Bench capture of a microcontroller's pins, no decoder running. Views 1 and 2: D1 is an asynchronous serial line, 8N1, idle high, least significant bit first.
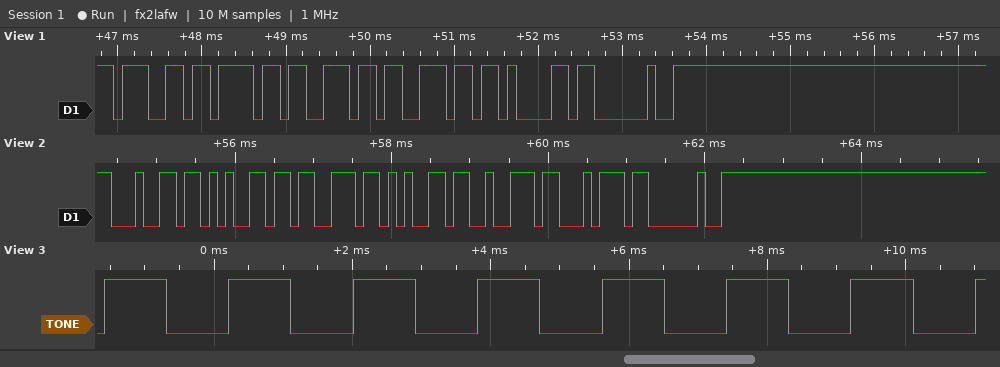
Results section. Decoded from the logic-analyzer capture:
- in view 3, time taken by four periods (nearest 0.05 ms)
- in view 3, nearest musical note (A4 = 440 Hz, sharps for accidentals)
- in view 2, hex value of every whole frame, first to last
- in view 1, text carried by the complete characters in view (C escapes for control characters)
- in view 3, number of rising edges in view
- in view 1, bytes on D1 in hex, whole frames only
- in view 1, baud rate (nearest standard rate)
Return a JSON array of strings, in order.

["7.20 ms", "C#5", "0x64 0x65 0x73 0x65 0x72 0x74 0x20", "\"gonna \"", "8", "67 6F 6E 6E 61 20", "9600 baud"]
